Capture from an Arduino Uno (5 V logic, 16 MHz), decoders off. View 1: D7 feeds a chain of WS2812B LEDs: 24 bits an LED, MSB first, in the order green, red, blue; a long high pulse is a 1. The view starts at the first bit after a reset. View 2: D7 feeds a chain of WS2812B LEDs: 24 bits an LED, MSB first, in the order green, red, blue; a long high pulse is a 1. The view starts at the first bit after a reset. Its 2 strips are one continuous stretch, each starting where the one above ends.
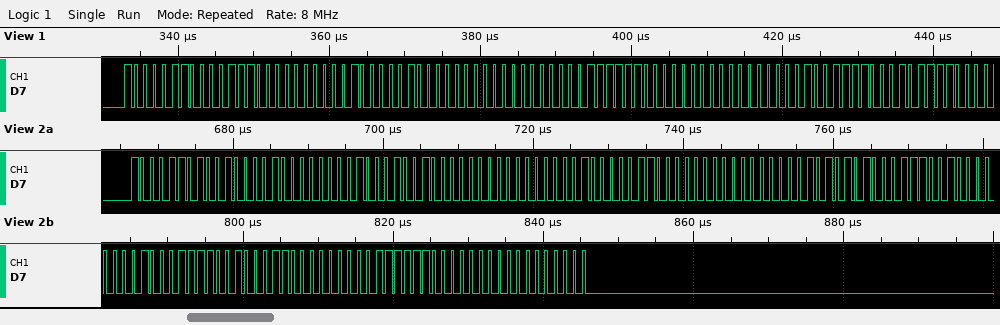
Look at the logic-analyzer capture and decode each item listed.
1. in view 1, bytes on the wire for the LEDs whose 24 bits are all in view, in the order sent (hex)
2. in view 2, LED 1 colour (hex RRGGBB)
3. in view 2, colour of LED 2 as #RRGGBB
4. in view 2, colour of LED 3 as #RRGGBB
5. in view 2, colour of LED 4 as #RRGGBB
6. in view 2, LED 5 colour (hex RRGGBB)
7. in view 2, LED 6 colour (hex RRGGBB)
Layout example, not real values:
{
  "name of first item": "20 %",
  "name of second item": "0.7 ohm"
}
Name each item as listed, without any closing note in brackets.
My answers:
{
  "in view 1, bytes on the wire for the LEDs whose 24 bits are all in view, in the order sent": "86 1C 00 82 00 00 7E 00 00",
  "in view 2, LED 1 colour": "#218D00",
  "in view 2, colour of LED 2 as #RRGGBB": "#008900",
  "in view 2, colour of LED 3 as #RRGGBB": "#008300",
  "in view 2, colour of LED 4 as #RRGGBB": "#39AA00",
  "in view 2, LED 5 colour": "#238F00",
  "in view 2, LED 6 colour": "#007E00"
}
